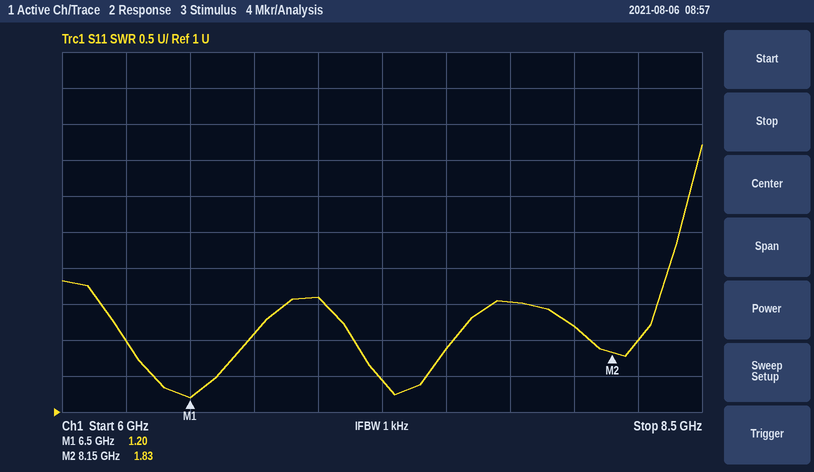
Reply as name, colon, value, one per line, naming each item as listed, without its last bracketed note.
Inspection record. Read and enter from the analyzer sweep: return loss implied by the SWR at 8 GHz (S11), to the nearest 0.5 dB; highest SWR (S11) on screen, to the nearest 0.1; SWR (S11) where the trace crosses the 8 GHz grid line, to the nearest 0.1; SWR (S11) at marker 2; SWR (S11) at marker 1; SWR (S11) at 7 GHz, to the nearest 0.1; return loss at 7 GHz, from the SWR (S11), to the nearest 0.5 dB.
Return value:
return loss implied by the SWR at 8 GHz (S11), to the nearest 0.5 dB: 8.5 dB
highest SWR (S11) on screen, to the nearest 0.1: 4.7
SWR (S11) where the trace crosses the 8 GHz grid line, to the nearest 0.1: 2.2
SWR (S11) at marker 2: 1.83
SWR (S11) at marker 1: 1.20
SWR (S11) at 7 GHz, to the nearest 0.1: 2.6
return loss at 7 GHz, from the SWR (S11), to the nearest 0.5 dB: 7.0 dB
